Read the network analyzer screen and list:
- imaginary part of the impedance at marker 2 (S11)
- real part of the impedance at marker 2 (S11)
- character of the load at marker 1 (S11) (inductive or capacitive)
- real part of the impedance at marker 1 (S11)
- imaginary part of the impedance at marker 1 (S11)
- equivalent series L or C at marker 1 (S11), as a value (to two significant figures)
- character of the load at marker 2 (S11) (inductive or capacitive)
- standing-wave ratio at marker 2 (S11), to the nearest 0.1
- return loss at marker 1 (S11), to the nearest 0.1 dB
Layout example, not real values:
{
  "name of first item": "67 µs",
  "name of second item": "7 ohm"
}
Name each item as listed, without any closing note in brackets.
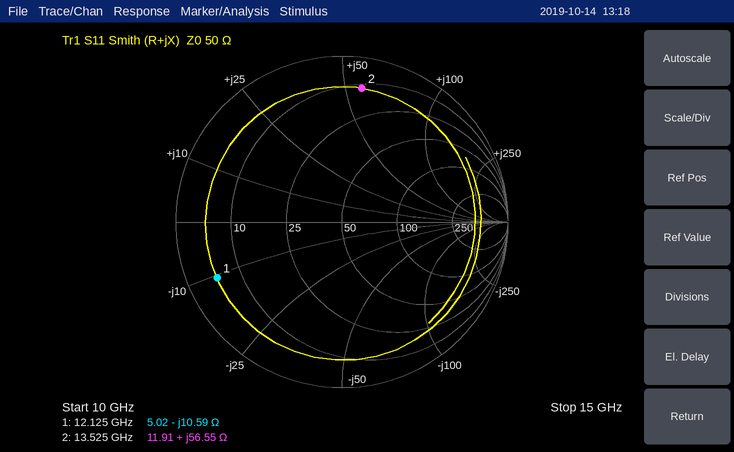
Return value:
{
  "imaginary part of the impedance at marker 2": "+56.55 Ω",
  "real part of the impedance at marker 2": "11.91 Ω",
  "character of the load at marker 1 (S11)": "capacitive",
  "real part of the impedance at marker 1": "5.02 Ω",
  "imaginary part of the impedance at marker 1": "-10.59 Ω",
  "equivalent series L or C at marker 1 (S11), as a value": "1.2 pF",
  "character of the load at marker 2 (S11)": "inductive",
  "standing-wave ratio at marker 2 (S11), to the nearest 0.1": "9.7",
  "return loss at marker 1 (S11), to the nearest 0.1 dB": "1.7 dB"
}
